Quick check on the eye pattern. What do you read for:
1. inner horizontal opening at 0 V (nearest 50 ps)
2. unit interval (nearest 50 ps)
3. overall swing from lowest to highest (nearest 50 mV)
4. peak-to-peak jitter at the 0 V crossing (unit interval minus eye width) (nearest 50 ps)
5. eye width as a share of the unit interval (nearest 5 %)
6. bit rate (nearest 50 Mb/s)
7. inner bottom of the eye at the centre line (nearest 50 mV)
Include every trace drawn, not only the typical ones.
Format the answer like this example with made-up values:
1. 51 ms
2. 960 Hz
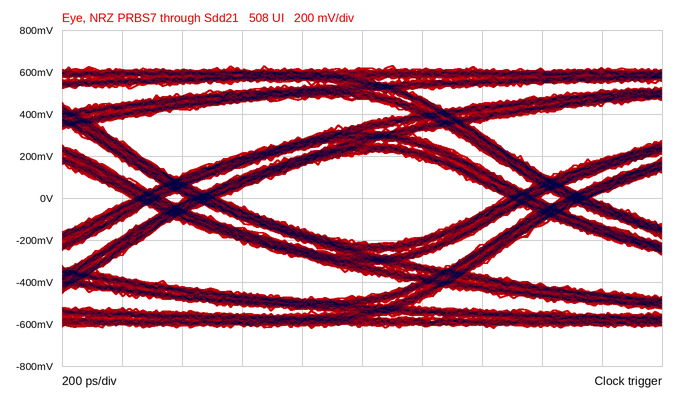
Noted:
1. 950 ps
2. 1.25 ns
3. 1.25 V
4. 300 ps
5. 75 %
6. 800 Mb/s
7. -200 mV
